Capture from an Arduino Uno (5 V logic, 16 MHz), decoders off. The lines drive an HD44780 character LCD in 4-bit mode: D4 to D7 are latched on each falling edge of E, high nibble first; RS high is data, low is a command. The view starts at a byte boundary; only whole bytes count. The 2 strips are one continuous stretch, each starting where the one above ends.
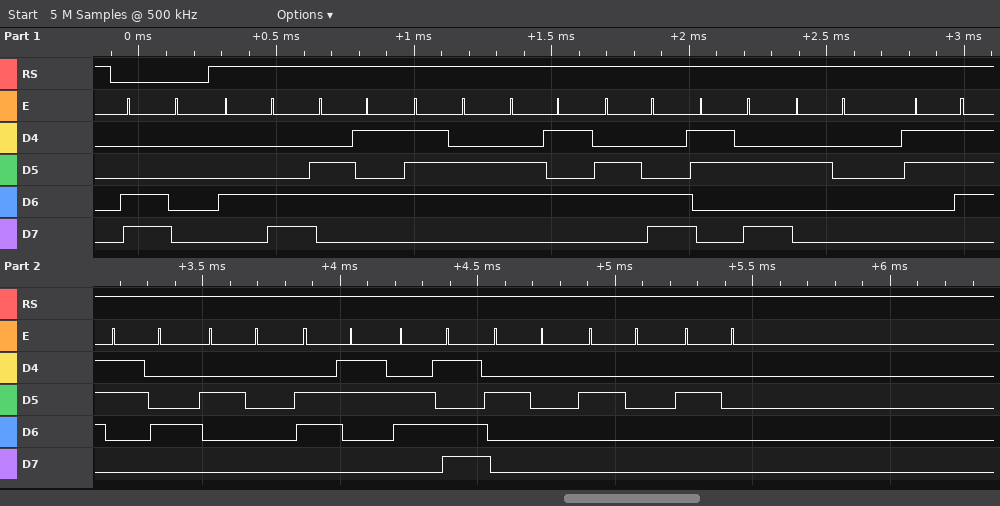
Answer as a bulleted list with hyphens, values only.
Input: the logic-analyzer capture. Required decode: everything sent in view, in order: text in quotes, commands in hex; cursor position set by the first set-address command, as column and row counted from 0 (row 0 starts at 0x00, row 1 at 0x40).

- 0xC0 "Level: 74 cm   "
- column 0, row 1
